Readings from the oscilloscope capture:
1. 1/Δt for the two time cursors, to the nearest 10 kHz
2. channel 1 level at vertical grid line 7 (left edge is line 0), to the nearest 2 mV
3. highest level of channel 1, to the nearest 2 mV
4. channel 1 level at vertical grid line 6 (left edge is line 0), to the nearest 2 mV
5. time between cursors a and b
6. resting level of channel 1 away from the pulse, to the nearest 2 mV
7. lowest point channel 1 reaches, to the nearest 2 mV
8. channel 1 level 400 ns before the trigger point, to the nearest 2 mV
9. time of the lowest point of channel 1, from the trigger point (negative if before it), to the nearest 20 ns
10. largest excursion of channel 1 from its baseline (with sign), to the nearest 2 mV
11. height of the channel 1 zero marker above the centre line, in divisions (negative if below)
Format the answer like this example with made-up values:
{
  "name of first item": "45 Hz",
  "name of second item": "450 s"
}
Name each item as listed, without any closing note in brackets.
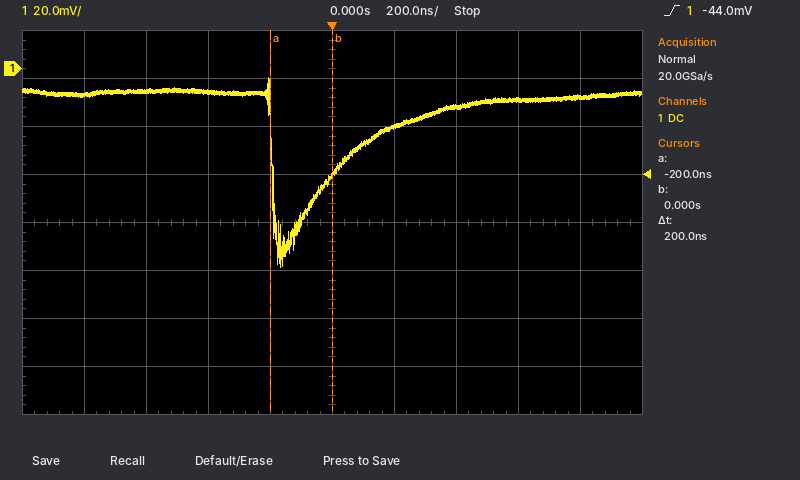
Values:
{
  "1/Δt for the two time cursors, to the nearest 10 kHz": "5.00 MHz",
  "channel 1 level at vertical grid line 7 (left edge is line 0), to the nearest 2 mV": "-16 mV",
  "highest level of channel 1, to the nearest 2 mV": "-4 mV",
  "channel 1 level at vertical grid line 6 (left edge is line 0), to the nearest 2 mV": "-24 mV",
  "time between cursors a and b": "200 ns",
  "resting level of channel 1 away from the pulse, to the nearest 2 mV": "-10 mV",
  "lowest point channel 1 reaches, to the nearest 2 mV": "-82 mV",
  "channel 1 level 400 ns before the trigger point, to the nearest 2 mV": "-10 mV",
  "time of the lowest point of channel 1, from the trigger point (negative if before it), to the nearest 20 ns": "-160 ns",
  "largest excursion of channel 1 from its baseline (with sign), to the nearest 2 mV": "-72 mV",
  "height of the channel 1 zero marker above the centre line, in divisions": "+3.2 div"
}
